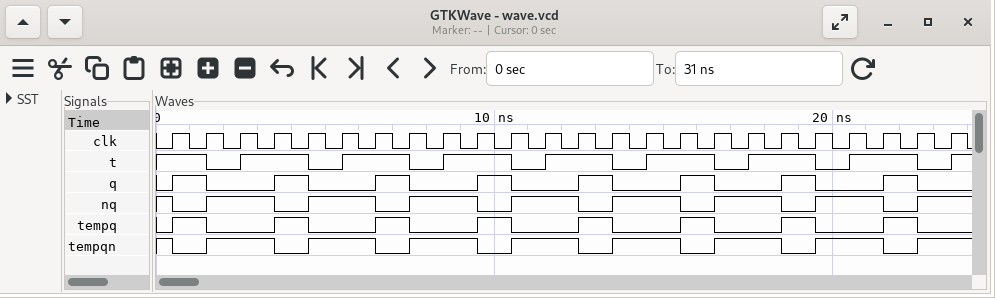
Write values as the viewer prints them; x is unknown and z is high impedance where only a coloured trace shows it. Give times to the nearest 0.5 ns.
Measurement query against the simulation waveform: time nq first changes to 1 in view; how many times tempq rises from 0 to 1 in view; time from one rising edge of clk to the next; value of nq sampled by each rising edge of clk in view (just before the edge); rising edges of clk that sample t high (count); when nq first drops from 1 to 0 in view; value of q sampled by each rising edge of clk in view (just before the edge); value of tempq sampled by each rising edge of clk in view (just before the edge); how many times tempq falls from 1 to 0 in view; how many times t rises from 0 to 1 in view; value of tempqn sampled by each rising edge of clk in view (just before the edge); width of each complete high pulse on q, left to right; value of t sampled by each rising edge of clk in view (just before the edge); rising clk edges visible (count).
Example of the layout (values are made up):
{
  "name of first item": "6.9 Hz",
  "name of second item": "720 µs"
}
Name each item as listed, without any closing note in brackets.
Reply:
{
  "time nq first changes to 1 in view": "1.5 ns",
  "how many times tempq rises from 0 to 1 in view": "8",
  "time from one rising edge of clk to the next": "1 ns",
  "value of nq sampled by each rising edge of clk in view": "1 0 1 1 0 1 1 0 1 1 0 1 1 0 1 1 0 1 1 0 1 1 0 1",
  "rising edges of clk that sample t high": "16",
  "when nq first drops from 1 to 0 in view": "0.5 ns",
  "value of q sampled by each rising edge of clk in view": "0 1 0 0 1 0 0 1 0 0 1 0 0 1 0 0 1 0 0 1 0 0 1 0",
  "value of tempq sampled by each rising edge of clk in view": "0 1 0 0 1 0 0 1 0 0 1 0 0 1 0 0 1 0 0 1 0 0 1 0",
  "how many times tempq falls from 1 to 0 in view": "8",
  "how many times t rises from 0 to 1 in view": "8",
  "value of tempqn sampled by each rising edge of clk in view": "1 0 1 1 0 1 1 0 1 1 0 1 1 0 1 1 0 1 1 0 1 1 0 1",
  "width of each complete high pulse on q, left to right": "1 ns, 1 ns, 1 ns, 1 ns, 1 ns, 1 ns, 1 ns, 1 ns",
  "value of t sampled by each rising edge of clk in view": "1 1 0 1 1 0 1 1 0 1 1 0 1 1 0 1 1 0 1 1 0 1 1 0",
  "rising clk edges visible": "24"
}
